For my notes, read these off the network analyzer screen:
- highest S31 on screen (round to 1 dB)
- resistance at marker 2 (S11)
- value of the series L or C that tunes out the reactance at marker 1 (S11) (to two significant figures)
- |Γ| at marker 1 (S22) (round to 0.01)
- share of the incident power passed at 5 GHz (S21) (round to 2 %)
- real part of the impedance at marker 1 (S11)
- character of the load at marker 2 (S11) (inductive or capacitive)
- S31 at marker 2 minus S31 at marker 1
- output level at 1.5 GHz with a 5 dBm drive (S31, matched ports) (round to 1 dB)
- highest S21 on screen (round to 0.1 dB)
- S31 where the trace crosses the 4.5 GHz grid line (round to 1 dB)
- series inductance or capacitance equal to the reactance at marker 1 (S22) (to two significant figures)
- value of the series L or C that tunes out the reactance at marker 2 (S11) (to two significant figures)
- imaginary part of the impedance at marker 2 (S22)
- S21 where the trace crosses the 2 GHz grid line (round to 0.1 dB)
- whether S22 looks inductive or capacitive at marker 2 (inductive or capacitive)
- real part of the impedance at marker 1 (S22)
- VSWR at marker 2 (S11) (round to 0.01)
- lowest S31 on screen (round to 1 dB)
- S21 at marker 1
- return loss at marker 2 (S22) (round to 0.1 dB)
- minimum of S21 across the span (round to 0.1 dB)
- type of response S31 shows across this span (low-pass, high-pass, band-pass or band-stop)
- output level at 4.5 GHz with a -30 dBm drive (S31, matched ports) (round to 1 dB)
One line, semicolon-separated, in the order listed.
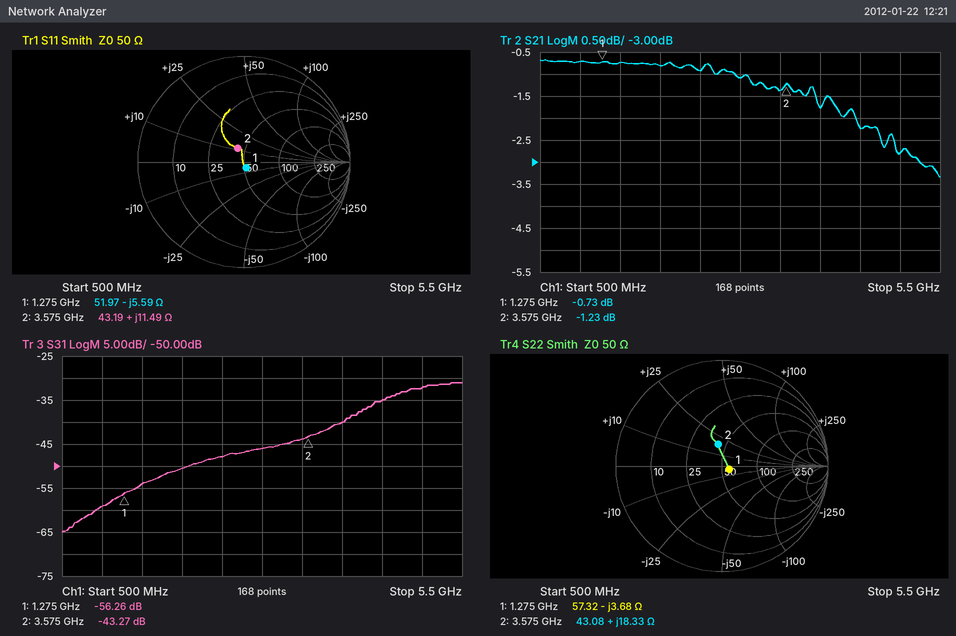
-31 dB; 43.19 Ω; 700 pH; 0.08; 52 %; 51.97 Ω; inductive; 12.99 dB; -49 dBm; -0.7 dB; -35 dB; 34 pF; 3.9 pF; +18.33 Ω; -0.8 dB; inductive; 57.32 Ω; 1.33; -65 dB; -0.73 dB; 13.7 dB; -3.3 dB; high-pass; -65 dBm
